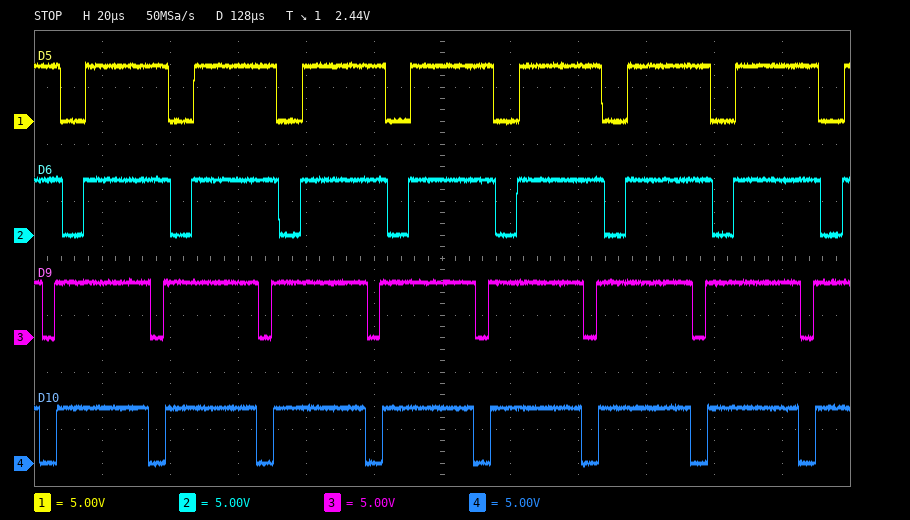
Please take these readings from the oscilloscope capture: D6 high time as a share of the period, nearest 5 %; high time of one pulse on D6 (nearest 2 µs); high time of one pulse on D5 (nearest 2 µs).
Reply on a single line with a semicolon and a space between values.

80 %; 26 µs; 24 µs
